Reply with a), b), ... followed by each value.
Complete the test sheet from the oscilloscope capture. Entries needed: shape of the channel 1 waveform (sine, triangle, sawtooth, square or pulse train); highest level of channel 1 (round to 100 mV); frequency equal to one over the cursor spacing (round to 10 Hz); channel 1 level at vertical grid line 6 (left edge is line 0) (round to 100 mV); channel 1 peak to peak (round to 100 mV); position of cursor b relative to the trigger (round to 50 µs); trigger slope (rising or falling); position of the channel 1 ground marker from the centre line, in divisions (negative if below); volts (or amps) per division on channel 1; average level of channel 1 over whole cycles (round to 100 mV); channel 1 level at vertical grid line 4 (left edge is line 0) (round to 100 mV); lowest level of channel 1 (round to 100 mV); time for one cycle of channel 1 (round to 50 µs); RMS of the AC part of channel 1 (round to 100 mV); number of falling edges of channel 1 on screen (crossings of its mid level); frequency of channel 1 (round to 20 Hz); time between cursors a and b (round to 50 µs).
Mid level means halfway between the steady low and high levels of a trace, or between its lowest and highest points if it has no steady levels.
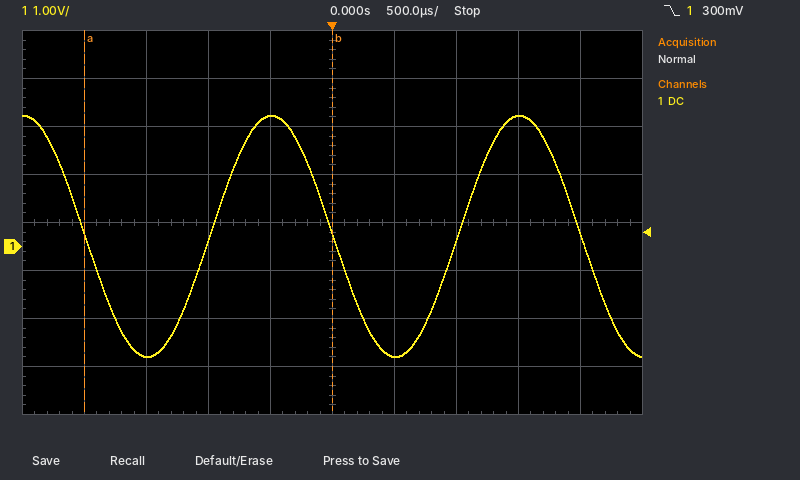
a) sine
b) 2.7 V
c) 500 Hz
d) -2.3 V
e) 5.0 V
f) 0 µs
g) falling
h) -0.5 div
i) 1 V
j) 200 mV
k) 2.7 V
l) -2.3 V
m) 2.00 ms
n) 1.8 V
o) 3
p) 500 Hz
q) 2.00 ms
